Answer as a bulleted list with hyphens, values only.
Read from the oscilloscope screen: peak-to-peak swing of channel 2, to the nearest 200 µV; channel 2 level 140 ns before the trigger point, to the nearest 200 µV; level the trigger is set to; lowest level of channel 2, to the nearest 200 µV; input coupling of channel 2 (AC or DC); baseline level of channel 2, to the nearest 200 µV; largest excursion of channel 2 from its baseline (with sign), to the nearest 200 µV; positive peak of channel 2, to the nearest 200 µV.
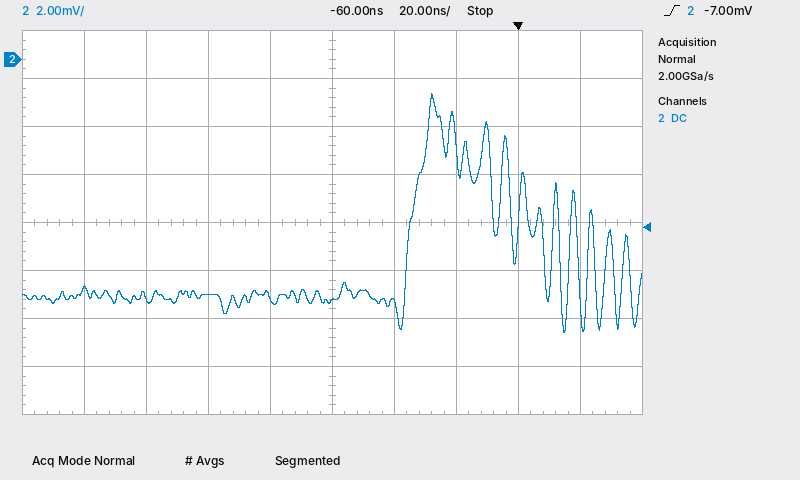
- 10.0 mV
- -9.6 mV
- -7.00 mV
- -11.4 mV
- DC
- -9.8 mV
- +8.4 mV
- -1.4 mV
